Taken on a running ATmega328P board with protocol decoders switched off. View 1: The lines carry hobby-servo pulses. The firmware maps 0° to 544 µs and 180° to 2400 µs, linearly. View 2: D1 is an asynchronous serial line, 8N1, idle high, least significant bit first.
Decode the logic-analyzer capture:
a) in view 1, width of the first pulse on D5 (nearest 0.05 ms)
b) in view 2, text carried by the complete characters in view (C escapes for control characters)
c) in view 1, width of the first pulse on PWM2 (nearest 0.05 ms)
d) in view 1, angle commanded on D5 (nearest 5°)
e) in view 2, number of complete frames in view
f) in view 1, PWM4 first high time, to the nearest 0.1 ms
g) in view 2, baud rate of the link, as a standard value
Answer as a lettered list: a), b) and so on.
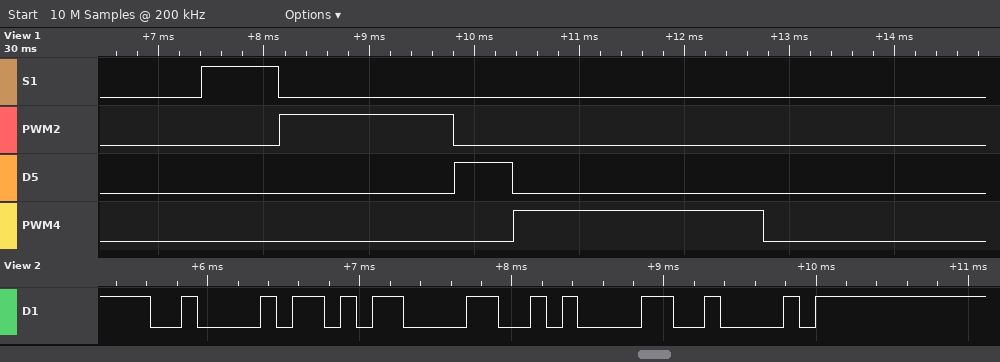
a) 0.55 ms
b) "B\r\nB"
c) 1.65 ms
d) 0°
e) 4
f) 2.4 ms
g) 9600 baud
